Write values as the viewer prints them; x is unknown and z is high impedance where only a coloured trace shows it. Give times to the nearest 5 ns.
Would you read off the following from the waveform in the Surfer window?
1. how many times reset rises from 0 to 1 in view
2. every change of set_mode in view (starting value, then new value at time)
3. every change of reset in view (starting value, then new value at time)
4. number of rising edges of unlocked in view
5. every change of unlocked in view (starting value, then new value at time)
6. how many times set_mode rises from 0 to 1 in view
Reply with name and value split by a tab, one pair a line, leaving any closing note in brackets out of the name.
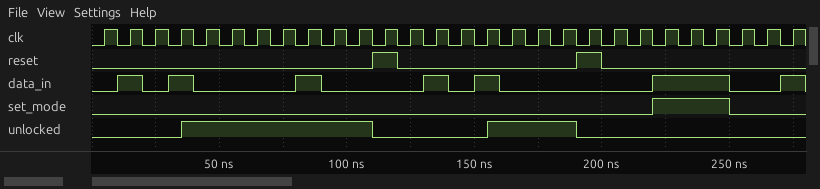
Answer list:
how many times reset rises from 0 to 1 in view	2
every change of set_mode in view	0, 1 at 220 ns, 0 at 250 ns
every change of reset in view	0, 1 at 110 ns, 0 at 120 ns, 1 at 190 ns, 0 at 200 ns
number of rising edges of unlocked in view	2
every change of unlocked in view	0, 1 at 35 ns, 0 at 110 ns, 1 at 155 ns, 0 at 190 ns
how many times set_mode rises from 0 to 1 in view	1
